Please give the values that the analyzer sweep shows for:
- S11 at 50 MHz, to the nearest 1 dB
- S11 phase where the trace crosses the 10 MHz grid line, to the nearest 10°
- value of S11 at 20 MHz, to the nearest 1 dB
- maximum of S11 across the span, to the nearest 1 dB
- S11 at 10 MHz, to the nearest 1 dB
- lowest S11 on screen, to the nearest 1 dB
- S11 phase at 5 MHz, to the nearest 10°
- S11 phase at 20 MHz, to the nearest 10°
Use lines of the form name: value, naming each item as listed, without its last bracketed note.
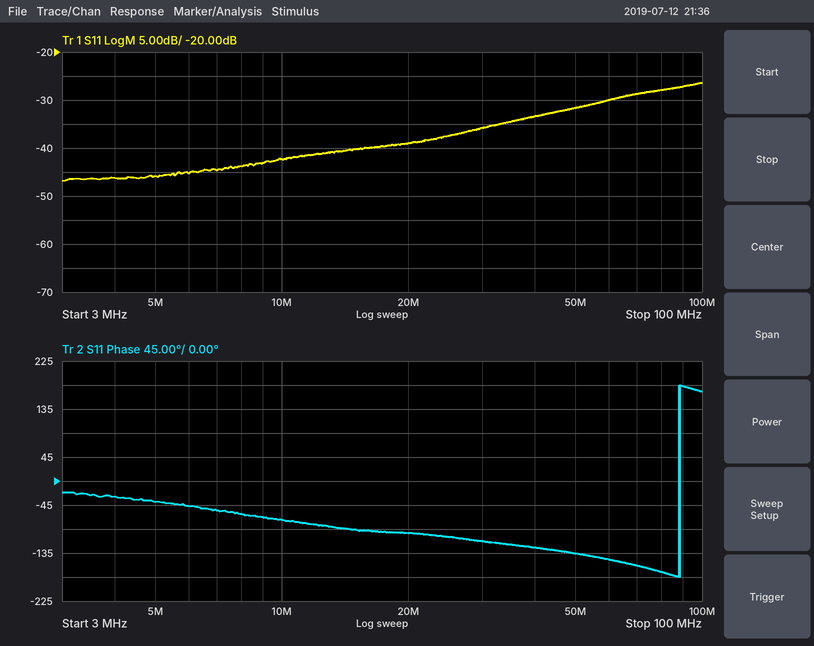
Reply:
S11 at 50 MHz, to the nearest 1 dB: -32 dB
S11 phase where the trace crosses the 10 MHz grid line, to the nearest 10°: -70°
value of S11 at 20 MHz, to the nearest 1 dB: -39 dB
maximum of S11 across the span, to the nearest 1 dB: -26 dB
S11 at 10 MHz, to the nearest 1 dB: -42 dB
lowest S11 on screen, to the nearest 1 dB: -47 dB
S11 phase at 5 MHz, to the nearest 10°: -40°
S11 phase at 20 MHz, to the nearest 10°: -100°
